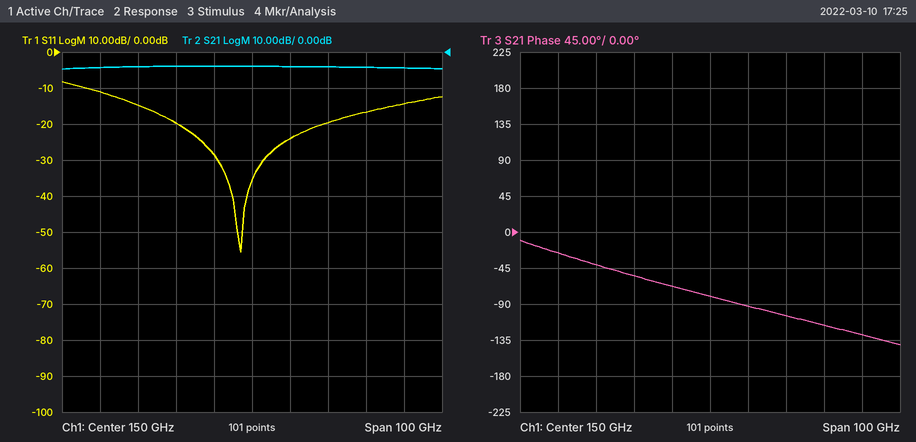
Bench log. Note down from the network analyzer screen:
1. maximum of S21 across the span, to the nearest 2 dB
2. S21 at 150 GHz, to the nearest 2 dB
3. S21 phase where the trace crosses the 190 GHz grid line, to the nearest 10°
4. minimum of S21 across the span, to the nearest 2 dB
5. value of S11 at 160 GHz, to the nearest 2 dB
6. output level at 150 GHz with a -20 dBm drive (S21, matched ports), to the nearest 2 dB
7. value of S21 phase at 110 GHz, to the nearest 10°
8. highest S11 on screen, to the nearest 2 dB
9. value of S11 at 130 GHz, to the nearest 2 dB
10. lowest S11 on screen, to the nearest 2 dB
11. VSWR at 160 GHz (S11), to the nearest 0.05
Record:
-4 dB
-4 dB
-130°
-4 dB
-24 dB
-24 dBm
-30°
-8 dB
-20 dB
-56 dB
1.15
